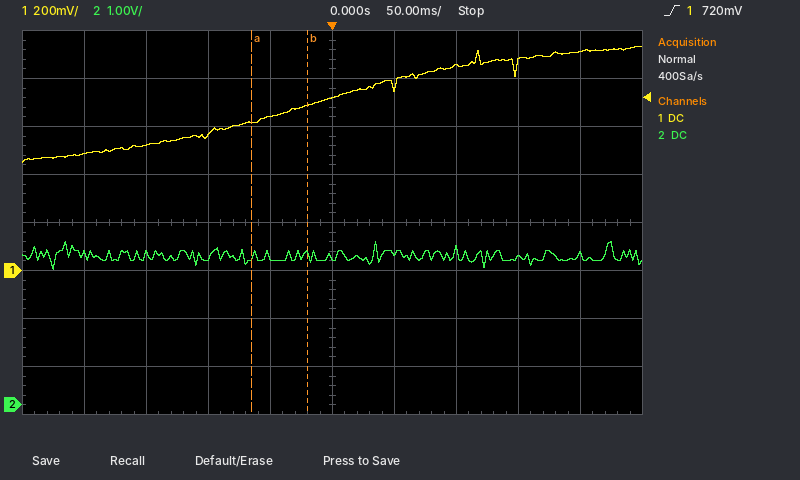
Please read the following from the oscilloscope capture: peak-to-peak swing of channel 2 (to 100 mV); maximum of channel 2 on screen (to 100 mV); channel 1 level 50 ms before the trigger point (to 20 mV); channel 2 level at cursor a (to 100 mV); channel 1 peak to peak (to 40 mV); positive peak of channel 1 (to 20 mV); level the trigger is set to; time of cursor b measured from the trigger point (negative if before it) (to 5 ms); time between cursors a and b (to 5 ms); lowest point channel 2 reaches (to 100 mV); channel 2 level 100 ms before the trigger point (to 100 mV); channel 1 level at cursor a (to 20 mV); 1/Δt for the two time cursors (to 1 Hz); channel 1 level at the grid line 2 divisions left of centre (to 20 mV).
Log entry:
600 mV
3.4 V
640 mV
3.1 V
480 mV
940 mV
720 mV
-20 ms
45 ms
2.8 V
3.1 V
620 mV
22 Hz
560 mV
